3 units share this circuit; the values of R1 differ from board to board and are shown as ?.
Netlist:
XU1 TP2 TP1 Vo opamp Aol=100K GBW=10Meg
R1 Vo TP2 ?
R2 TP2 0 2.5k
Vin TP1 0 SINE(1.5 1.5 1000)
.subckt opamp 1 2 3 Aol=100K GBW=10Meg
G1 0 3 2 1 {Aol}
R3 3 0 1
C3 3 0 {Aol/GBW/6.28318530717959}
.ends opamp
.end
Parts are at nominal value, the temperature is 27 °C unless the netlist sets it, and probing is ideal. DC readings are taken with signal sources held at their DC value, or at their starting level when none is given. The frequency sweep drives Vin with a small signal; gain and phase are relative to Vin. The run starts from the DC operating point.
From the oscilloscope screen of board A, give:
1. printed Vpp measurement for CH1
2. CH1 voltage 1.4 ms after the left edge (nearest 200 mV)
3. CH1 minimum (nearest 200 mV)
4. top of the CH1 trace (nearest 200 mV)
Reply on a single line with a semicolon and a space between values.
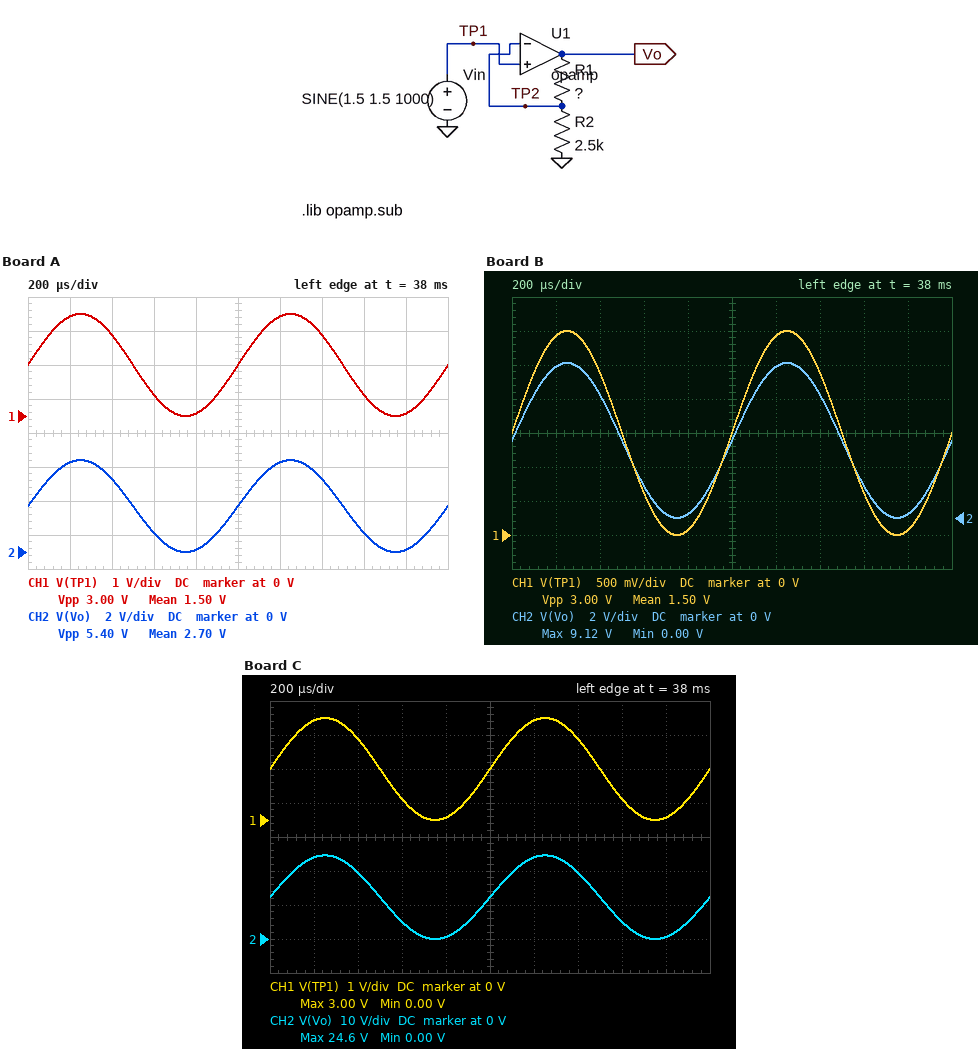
3.00 V; 2.4 V; 0 V; 3.0 V
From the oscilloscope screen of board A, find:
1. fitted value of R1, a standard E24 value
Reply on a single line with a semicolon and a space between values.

2 kΩ
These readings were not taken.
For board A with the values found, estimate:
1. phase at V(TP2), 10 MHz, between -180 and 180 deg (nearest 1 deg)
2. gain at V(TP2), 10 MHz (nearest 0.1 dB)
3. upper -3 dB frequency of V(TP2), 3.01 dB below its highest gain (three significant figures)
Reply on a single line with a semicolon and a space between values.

-61 deg; -6.3 dB; 5.56 MHz
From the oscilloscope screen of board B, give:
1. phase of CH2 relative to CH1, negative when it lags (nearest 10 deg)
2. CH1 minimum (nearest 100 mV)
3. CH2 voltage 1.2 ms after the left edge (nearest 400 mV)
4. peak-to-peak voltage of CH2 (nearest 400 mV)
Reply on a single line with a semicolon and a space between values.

0 deg; 0 V; 8.8 V; 9.2 V
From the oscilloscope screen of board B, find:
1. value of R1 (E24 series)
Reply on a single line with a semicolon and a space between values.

5.1 kΩ
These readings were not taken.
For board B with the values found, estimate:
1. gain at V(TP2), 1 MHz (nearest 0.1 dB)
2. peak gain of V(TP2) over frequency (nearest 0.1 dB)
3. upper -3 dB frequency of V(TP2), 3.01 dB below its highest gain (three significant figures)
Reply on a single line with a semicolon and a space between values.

-0.4 dB; 0 dB; 3.29 MHz
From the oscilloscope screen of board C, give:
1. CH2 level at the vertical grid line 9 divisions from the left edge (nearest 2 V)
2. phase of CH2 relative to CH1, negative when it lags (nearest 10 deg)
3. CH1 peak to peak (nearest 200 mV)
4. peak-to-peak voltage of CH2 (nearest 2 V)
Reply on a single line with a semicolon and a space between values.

0 V; 0 deg; 3.0 V; 24 V
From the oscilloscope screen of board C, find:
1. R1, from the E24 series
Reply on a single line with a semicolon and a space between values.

18 kΩ
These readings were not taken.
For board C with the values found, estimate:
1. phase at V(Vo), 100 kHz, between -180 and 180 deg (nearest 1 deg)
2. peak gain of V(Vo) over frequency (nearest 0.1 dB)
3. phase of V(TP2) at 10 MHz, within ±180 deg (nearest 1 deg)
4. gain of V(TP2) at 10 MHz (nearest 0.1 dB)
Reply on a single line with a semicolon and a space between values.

-5 deg; 18.3 dB; -83 deg; -18.3 dB
